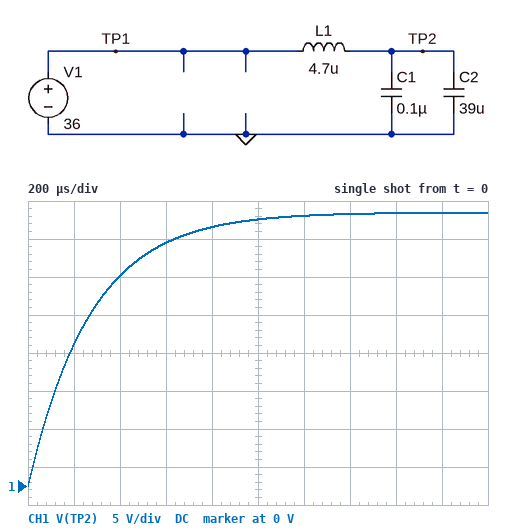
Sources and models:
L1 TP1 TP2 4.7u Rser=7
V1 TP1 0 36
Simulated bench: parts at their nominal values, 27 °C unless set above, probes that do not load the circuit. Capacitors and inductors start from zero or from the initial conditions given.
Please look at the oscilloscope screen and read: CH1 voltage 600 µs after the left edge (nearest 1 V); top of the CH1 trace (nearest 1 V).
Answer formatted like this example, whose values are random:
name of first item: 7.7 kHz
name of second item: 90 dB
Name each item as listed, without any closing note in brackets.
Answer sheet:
CH1 voltage 600 µs after the left edge: 32 V
top of the CH1 trace: 36 V
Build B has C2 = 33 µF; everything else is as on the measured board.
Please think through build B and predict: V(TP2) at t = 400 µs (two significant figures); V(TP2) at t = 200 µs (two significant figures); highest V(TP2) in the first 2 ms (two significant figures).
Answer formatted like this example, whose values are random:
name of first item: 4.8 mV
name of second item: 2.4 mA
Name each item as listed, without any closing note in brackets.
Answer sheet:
V(TP2) at t = 400 µs: 30 V
V(TP2) at t = 200 µs: 21 V
highest V(TP2) in the first 2 ms: 36 V
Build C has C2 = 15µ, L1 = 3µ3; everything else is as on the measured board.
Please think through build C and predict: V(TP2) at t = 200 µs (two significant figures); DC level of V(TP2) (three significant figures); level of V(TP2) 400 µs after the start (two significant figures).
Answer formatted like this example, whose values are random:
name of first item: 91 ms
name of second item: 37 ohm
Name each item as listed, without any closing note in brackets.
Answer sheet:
V(TP2) at t = 200 µs: 31 V
DC level of V(TP2): 36.0 V
level of V(TP2) 400 µs after the start: 35 V
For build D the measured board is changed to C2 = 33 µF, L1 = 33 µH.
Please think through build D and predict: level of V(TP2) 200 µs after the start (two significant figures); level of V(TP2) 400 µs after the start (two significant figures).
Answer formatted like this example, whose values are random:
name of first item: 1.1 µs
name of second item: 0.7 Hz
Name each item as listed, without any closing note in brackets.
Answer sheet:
level of V(TP2) 200 µs after the start: 21 V
level of V(TP2) 400 µs after the start: 30 V
